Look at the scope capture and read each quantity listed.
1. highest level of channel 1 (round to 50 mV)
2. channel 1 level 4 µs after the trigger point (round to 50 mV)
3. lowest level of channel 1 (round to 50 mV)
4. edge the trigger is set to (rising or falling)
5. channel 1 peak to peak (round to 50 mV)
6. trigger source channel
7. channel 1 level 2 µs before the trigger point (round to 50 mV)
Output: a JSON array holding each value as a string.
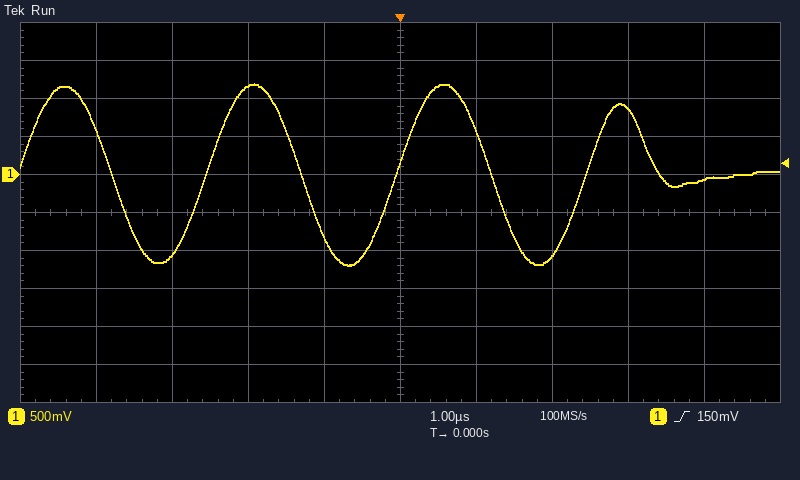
["1.20 V", "-50 mV", "-1.20 V", "rising", "2.40 V", "channel 1", "1.15 V"]
